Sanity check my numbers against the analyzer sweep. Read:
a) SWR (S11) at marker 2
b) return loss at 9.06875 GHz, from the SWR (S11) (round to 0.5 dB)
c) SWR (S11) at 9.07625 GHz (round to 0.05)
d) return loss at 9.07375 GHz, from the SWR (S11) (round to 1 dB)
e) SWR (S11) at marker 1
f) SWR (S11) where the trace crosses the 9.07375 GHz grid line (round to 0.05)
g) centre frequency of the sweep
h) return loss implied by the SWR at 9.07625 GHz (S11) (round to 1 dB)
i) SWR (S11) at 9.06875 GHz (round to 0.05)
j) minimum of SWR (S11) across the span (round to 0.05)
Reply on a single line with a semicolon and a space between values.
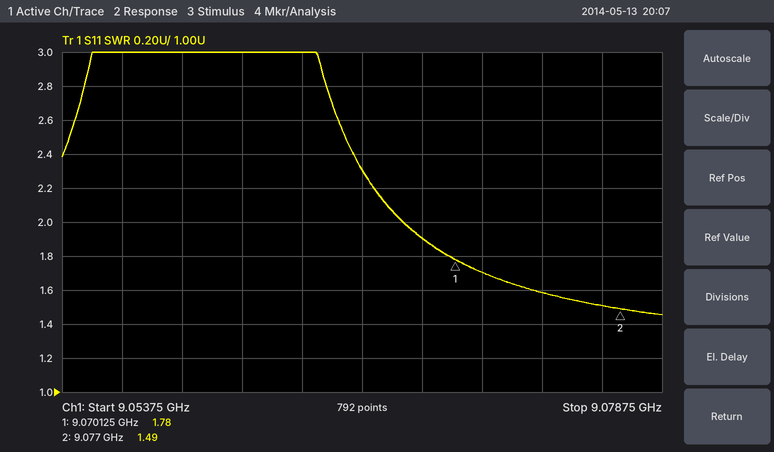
1.49; 10.0 dB; 1.50; 13 dB; 1.78; 1.60; 9.06625 GHz; 14 dB; 1.90; 1.45
